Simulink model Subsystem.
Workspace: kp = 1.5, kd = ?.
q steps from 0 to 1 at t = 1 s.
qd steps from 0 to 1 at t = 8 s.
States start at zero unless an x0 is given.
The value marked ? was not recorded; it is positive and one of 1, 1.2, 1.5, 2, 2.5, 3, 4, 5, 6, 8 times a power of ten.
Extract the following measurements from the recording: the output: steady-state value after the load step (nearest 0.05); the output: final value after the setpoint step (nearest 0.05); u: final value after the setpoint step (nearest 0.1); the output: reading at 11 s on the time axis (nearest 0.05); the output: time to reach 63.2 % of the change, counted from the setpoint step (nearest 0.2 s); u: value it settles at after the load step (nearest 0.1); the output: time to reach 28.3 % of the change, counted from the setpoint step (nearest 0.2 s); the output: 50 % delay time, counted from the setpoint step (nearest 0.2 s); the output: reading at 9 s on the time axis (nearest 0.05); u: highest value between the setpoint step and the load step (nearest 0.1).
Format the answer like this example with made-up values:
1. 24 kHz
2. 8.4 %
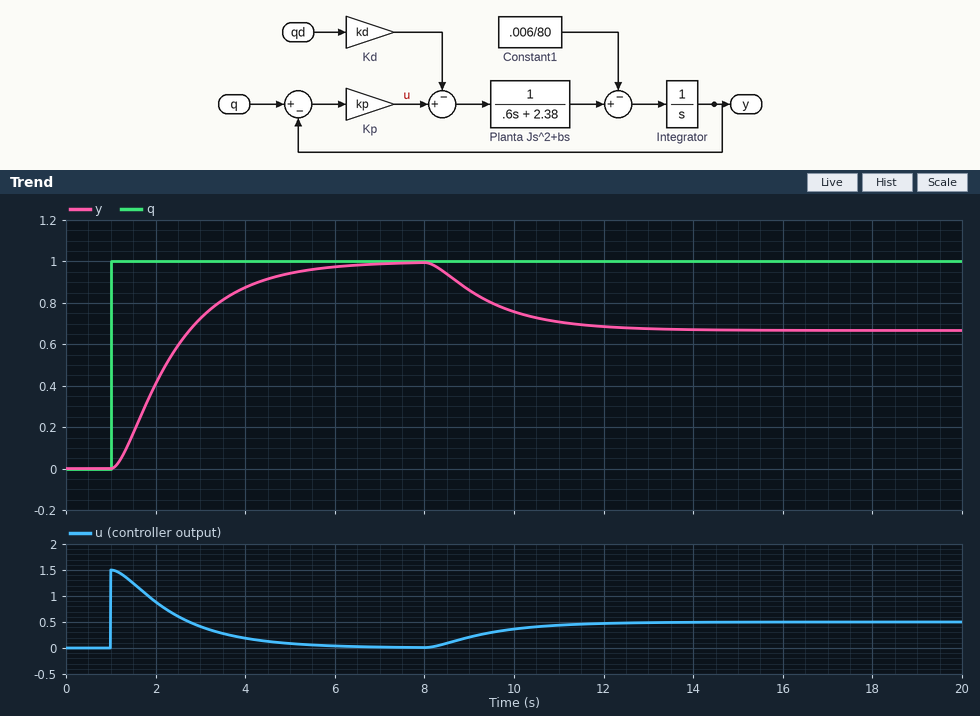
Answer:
1. 0.65
2. 1.00
3. 0.0
4. 0.70
5. 1.6 s
6. 0.5
7. 0.8 s
8. 1.2 s
9. 0.85
10. 1.5
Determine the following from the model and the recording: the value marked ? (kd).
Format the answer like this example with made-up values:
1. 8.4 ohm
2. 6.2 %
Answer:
1. 0.5
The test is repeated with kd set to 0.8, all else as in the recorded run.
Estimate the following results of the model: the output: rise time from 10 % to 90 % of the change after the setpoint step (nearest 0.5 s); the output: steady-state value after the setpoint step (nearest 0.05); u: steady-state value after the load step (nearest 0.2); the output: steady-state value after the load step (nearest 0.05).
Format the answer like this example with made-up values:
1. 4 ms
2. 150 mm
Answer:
1. 3.0 s
2. 1.00
3. 0.8
4. 0.45
